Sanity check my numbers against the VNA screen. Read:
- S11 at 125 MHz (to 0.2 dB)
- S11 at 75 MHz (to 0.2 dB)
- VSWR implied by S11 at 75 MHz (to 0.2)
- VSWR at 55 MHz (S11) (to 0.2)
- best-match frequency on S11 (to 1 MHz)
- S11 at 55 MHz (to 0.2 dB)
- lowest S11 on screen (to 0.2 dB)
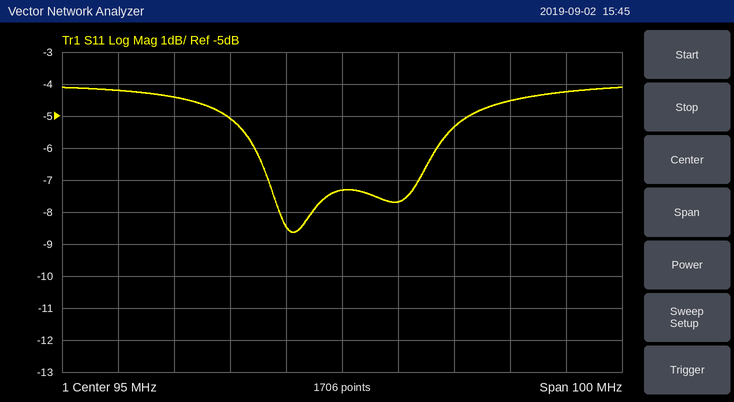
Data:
-4.6 dB
-5.0 dB
3.6
4.2
86 MHz
-4.2 dB
-8.6 dB
